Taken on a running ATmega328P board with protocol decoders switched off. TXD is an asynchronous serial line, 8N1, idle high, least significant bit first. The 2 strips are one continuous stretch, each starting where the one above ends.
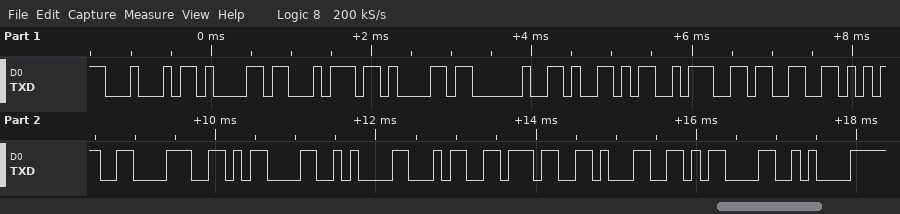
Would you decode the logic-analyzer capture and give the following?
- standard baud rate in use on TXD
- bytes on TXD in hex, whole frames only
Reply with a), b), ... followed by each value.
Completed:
a) 9600 baud
b) 44 61 74 61 20 59 3A 33 35 38 0D 0A 34 37 31 0D 0A
